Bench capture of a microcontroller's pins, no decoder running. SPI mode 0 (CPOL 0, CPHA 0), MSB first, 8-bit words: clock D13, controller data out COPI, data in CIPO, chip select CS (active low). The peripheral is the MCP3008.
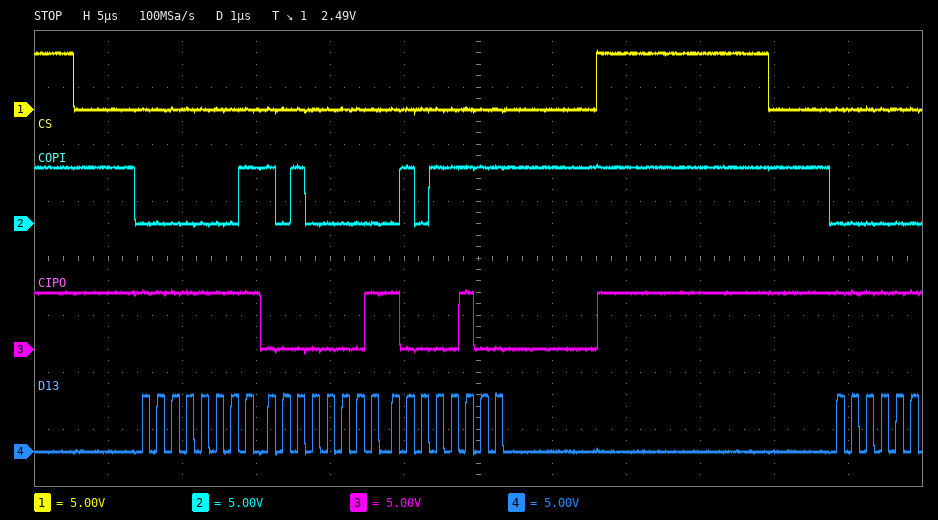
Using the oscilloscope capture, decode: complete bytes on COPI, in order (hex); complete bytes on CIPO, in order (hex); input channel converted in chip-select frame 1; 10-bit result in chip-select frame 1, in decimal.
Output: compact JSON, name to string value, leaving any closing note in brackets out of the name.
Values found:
{"complete bytes on COPI, in order": "01 A0 5F", "complete bytes on CIPO, in order": "FF 01 84", "input channel converted in chip-select frame 1": "2", "10-bit result in chip-select frame 1, in decimal": "388"}
